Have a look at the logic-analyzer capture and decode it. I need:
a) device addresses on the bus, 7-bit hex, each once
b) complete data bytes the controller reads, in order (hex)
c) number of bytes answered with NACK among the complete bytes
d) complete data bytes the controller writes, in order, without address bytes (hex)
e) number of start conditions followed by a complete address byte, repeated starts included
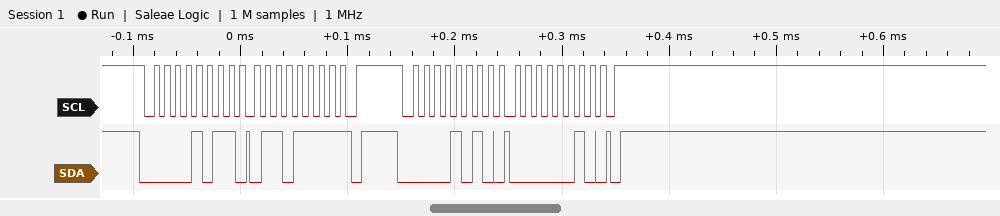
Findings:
0x05
6F
1
02
2
